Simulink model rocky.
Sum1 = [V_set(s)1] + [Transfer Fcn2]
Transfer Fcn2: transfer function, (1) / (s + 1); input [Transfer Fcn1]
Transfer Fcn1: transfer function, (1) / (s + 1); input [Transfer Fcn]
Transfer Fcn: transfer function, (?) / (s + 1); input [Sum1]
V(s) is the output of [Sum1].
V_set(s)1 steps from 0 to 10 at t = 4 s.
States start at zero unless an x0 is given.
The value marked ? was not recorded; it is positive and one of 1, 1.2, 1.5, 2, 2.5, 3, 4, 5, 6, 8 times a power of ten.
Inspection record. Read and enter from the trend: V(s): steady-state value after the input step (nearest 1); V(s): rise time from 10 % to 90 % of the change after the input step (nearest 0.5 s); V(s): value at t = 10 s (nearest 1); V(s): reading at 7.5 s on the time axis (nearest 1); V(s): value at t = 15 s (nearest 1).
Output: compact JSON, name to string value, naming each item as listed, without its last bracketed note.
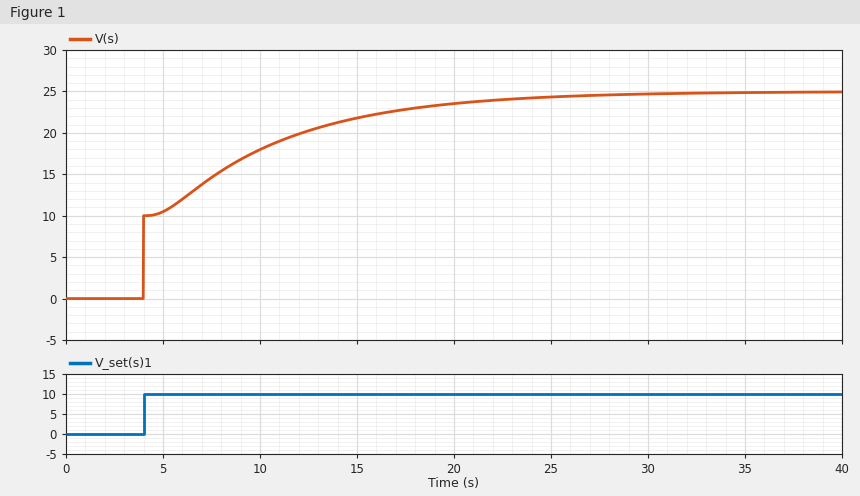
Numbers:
{"V(s): steady-state value after the input step": "25", "V(s): rise time from 10 % to 90 % of the change after the input step": "12.5 s", "V(s): value at t = 10 s": "18", "V(s): reading at 7.5 s on the time axis": "15", "V(s): value at t = 15 s": "22"}
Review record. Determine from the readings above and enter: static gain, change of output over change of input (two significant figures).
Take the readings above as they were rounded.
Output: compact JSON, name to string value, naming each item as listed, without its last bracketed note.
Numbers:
{"static gain, change of output over change of input": "2.5"}
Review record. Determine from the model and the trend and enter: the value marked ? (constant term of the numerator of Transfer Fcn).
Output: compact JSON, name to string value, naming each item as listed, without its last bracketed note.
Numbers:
{"the value marked ?": "0.6"}
